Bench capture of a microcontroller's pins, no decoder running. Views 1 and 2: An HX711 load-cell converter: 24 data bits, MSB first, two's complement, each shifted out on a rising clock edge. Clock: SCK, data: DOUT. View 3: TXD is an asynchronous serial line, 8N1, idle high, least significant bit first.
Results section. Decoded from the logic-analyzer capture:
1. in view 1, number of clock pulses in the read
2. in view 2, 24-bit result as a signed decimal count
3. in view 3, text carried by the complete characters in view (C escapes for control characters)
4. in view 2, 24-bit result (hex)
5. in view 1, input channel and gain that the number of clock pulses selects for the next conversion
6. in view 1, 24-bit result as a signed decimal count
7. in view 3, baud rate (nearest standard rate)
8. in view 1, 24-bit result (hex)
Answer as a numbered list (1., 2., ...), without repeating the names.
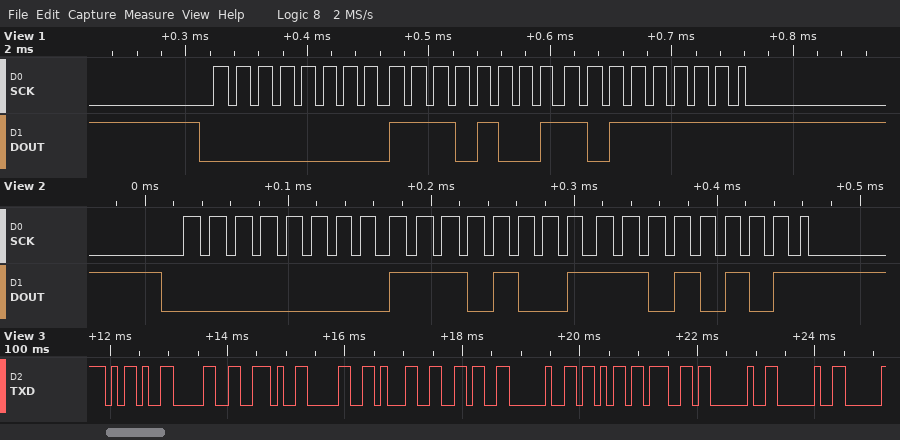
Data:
1. 25
2. 59861
3. "-0.016 kg  "
4. 0x00E9D5
5. channel A, gain 128
6. 59839
7. 9600 baud
8. 0x00E9BF
